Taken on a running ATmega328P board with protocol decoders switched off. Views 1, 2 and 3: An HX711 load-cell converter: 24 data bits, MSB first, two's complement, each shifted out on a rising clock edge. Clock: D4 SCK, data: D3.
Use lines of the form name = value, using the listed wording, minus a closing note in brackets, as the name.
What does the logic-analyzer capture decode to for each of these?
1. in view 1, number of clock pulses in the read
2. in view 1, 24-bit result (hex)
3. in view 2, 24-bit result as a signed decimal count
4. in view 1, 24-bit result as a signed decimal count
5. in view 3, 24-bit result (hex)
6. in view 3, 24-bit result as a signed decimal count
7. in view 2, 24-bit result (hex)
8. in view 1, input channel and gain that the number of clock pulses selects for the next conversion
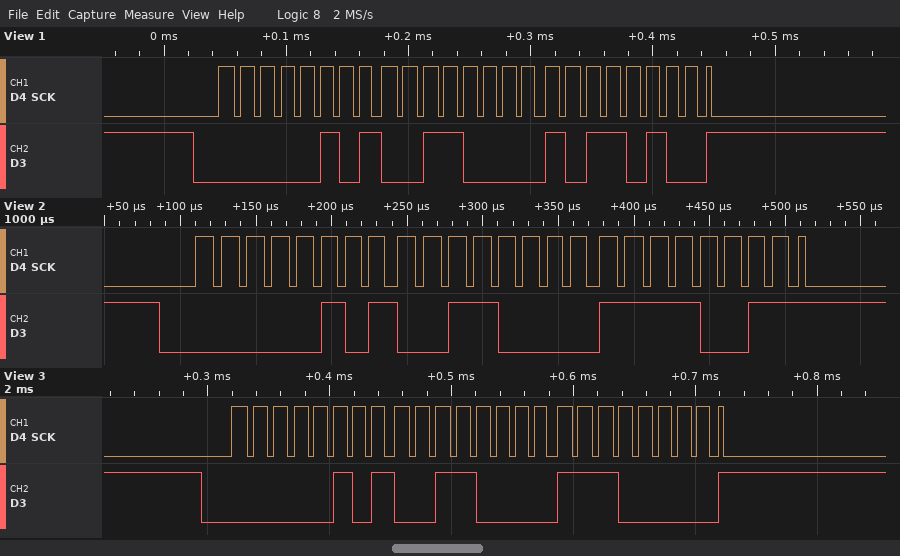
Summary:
in view 1, number of clock pulses in the read = 25
in view 1, 24-bit result = 0x0530B4
in view 2, 24-bit result as a signed decimal count = 340211
in view 1, 24-bit result as a signed decimal count = 340148
in view 3, 24-bit result = 0x0530E0
in view 3, 24-bit result as a signed decimal count = 340192
in view 2, 24-bit result = 0x0530F3
in view 1, input channel and gain that the number of clock pulses selects for the next conversion = channel A, gain 128
